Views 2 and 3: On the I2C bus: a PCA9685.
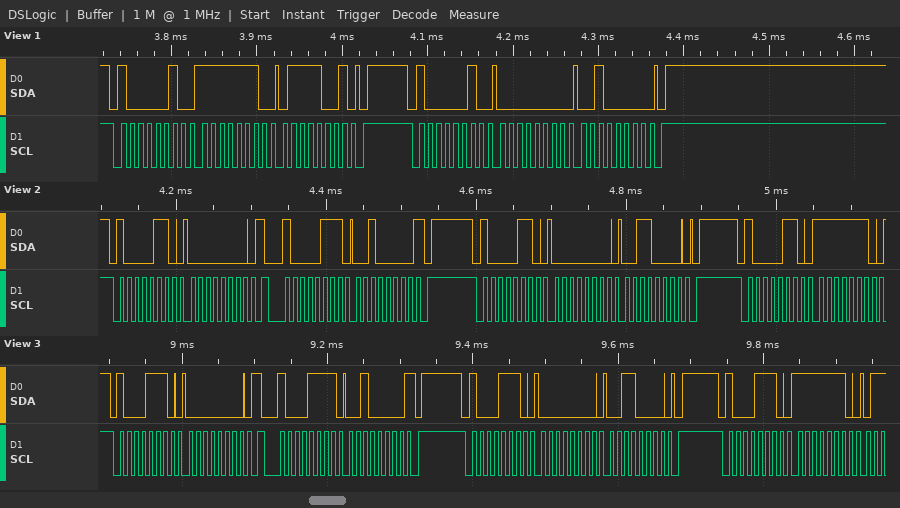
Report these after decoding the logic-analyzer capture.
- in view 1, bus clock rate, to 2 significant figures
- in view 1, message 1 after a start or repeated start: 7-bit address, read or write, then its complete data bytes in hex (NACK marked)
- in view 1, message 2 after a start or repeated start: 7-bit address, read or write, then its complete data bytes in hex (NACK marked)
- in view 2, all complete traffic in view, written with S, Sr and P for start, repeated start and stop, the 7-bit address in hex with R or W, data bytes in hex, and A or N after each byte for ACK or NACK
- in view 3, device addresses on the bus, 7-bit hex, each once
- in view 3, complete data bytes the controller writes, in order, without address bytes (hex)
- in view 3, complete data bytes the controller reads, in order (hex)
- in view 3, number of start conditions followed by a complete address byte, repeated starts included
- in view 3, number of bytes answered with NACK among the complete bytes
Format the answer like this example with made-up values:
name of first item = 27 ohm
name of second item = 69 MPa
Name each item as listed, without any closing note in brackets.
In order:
in view 1, bus clock rate, to 2 significant figures = 100 kHz
in view 1, message 1 after a start or repeated start: 7-bit address, read or write, then its complete data bytes in hex = 0x41 write: FE 79
in view 1, message 2 after a start or repeated start: 7-bit address, read or write, then its complete data bytes in hex = 0x41 write: 00 20
in view 2, all complete traffic in view, written with S, Sr and P for start, repeated start and stop, the 7-bit address in hex with R or W, data bytes in hex, and A or N after each byte for ACK or NACK = S 43W A 00 A Sr 43R A 20 N P S 43W A 00 A 30 A P S 43W A FE A
in view 3, device addresses on the bus, 7-bit hex, each once = 0x47
in view 3, complete data bytes the controller writes, in order, without address bytes = 00 00 30 FE
in view 3, complete data bytes the controller reads, in order = 20
in view 3, number of start conditions followed by a complete address byte, repeated starts included = 4
in view 3, number of bytes answered with NACK among the complete bytes = 1
